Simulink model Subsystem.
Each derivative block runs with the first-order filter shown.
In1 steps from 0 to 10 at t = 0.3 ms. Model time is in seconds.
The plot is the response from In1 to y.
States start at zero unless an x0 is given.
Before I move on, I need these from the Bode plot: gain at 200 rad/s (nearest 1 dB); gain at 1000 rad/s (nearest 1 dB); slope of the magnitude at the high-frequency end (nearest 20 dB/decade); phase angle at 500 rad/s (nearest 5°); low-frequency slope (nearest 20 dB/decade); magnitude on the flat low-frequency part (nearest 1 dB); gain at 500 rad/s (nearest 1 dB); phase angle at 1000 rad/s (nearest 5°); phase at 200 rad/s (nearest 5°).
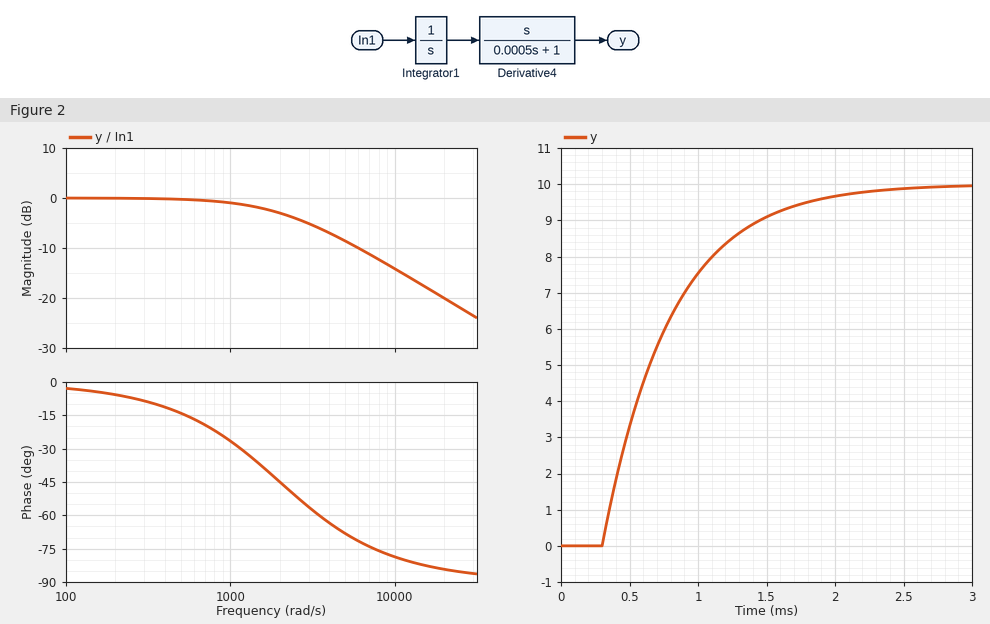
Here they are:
0 dB
-1 dB
-20 dB/decade
-15°
0 dB/decade
0 dB
0 dB
-25°
-5°
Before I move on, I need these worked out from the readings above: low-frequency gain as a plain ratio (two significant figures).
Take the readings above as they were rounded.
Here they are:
1.0
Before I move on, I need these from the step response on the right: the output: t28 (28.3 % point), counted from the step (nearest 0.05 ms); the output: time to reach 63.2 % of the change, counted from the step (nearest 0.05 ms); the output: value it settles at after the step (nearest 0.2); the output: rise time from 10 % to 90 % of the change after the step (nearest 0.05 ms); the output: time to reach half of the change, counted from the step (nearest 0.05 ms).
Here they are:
0.15 ms
0.50 ms
10.0
1.10 ms
0.35 ms
